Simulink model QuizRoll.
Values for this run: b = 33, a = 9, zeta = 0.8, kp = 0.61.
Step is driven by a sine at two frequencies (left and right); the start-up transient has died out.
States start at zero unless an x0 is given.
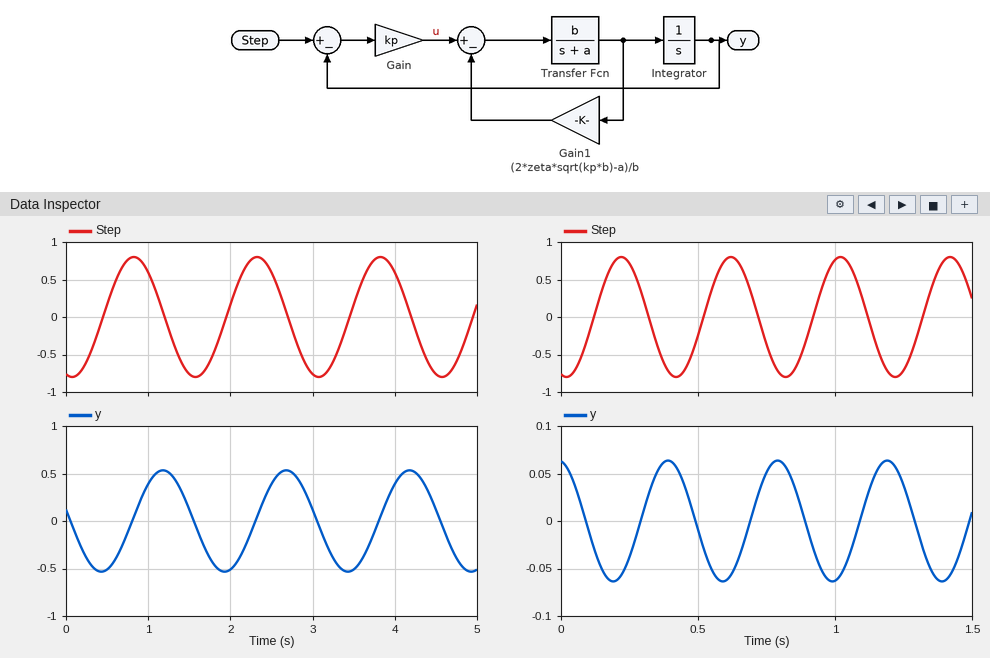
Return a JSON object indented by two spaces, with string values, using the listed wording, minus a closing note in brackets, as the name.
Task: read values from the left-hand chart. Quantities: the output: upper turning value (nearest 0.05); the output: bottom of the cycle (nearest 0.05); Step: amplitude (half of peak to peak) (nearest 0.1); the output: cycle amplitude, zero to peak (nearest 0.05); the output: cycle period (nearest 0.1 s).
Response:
{
  "the output: upper turning value": "0.55",
  "the output: bottom of the cycle": "-0.55",
  "Step: amplitude (half of peak to peak)": "0.8",
  "the output: cycle amplitude, zero to peak": "0.55",
  "the output: cycle period": "1.5 s"
}
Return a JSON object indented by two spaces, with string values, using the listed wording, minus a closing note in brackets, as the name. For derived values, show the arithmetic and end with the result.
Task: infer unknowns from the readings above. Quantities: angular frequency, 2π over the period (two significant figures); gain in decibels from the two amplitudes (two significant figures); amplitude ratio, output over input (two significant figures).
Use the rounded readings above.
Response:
{
  "angular frequency, 2π over the period": "2π / 1.5 = 4.2 rad/s",
  "gain in decibels from the two amplitudes": "20 log10(0.55 / 0.8) = -3.3 dB",
  "amplitude ratio, output over input": "0.55 / 0.8 = 0.69"
}
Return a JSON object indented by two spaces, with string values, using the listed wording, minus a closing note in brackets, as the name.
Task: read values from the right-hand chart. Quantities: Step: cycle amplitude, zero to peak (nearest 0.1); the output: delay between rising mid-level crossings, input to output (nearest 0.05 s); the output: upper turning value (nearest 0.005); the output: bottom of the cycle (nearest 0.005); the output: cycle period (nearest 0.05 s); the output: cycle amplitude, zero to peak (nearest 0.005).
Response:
{
  "Step: cycle amplitude, zero to peak": "0.8",
  "the output: delay between rising mid-level crossings, input to output": "0.15 s",
  "the output: upper turning value": "0.065",
  "the output: bottom of the cycle": "-0.065",
  "the output: cycle period": "0.40 s",
  "the output: cycle amplitude, zero to peak": "0.065"
}
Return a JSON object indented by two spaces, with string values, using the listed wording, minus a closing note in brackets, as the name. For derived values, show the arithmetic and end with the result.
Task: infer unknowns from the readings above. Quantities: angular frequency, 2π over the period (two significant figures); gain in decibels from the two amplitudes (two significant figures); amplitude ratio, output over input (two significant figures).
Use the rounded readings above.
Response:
{
  "angular frequency, 2π over the period": "2π / 0.4 = 16 rad/s",
  "gain in decibels from the two amplitudes": "20 log10(0.065 / 0.8) = -22 dB",
  "amplitude ratio, output over input": "0.065 / 0.8 = 0.081"
}
